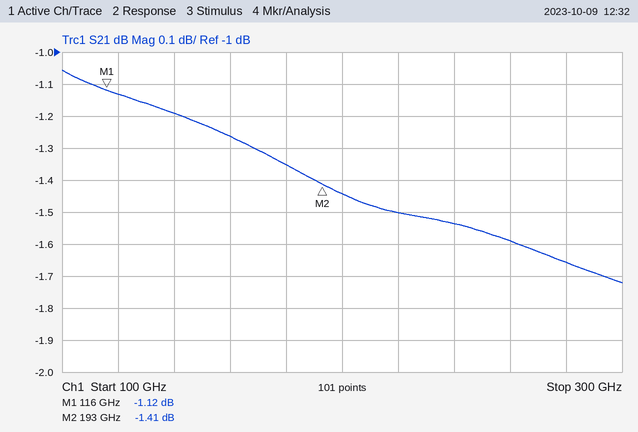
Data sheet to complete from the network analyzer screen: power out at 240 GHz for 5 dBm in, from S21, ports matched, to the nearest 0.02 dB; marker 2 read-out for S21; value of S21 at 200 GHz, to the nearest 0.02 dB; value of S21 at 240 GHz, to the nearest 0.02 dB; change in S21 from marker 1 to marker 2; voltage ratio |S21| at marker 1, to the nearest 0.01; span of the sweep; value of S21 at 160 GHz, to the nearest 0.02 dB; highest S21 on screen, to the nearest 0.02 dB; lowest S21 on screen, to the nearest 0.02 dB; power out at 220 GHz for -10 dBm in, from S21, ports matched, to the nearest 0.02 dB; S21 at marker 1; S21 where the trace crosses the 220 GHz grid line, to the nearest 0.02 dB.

3.46 dBm
-1.41 dB
-1.44 dB
-1.54 dB
-0.29 dB
0.88
200 GHz
-1.26 dB
-1.06 dB
-1.72 dB
-11.50 dBm
-1.12 dB
-1.50 dB
